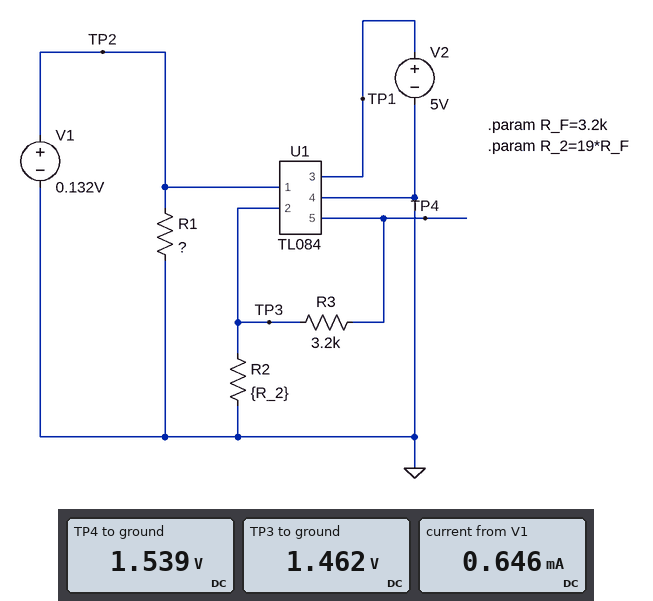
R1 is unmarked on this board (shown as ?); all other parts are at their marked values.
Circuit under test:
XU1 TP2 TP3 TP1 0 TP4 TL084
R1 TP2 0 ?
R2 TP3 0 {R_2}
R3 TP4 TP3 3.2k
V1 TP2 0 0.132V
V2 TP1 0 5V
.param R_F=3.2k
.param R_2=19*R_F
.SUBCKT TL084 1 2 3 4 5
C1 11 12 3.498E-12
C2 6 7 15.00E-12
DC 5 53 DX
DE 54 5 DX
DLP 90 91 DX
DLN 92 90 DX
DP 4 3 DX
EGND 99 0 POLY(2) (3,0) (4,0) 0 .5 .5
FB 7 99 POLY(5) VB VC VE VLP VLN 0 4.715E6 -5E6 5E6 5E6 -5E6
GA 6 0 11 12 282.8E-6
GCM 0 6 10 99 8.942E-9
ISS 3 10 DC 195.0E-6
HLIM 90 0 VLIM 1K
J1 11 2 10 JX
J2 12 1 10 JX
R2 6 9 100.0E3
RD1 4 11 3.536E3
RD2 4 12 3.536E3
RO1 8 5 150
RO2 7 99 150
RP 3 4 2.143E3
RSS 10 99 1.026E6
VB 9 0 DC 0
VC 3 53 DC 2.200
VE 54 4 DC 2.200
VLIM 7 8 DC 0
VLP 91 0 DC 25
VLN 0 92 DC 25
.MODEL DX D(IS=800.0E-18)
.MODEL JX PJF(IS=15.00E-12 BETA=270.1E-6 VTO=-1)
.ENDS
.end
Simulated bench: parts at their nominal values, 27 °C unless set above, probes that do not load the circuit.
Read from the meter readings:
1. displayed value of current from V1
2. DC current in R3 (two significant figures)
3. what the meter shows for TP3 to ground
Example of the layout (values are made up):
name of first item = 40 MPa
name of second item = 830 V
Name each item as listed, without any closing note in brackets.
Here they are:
displayed value of current from V1 = 0.646 mA
DC current in R3 = 24 µA
what the meter shows for TP3 to ground = 1.462 V
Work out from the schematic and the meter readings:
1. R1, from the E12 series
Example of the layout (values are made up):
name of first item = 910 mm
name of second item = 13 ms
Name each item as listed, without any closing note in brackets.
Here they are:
R1, from the E12 series = 180 Ω
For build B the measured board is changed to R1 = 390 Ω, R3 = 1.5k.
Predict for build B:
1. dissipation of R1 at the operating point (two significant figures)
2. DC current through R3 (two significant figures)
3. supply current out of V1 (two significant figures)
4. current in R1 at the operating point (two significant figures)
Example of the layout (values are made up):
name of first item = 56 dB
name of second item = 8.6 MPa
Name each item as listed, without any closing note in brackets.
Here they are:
dissipation of R1 at the operating point = 45 µW
DC current through R3 = 25 µA
supply current out of V1 = 250 µA
current in R1 at the operating point = 340 µA
